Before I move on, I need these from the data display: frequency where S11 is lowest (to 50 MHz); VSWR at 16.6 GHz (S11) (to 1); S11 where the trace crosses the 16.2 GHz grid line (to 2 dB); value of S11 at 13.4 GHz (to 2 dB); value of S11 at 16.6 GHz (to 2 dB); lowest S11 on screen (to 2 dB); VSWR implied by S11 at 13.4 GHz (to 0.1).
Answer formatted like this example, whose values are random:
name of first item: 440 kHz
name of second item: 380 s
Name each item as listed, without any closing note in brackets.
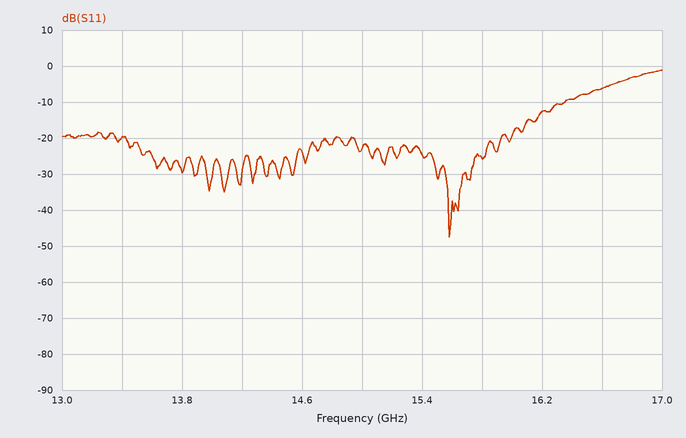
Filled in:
frequency where S11 is lowest: 15.60 GHz
VSWR at 16.6 GHz (S11): 3
S11 where the trace crosses the 16.2 GHz grid line: -12 dB
value of S11 at 13.4 GHz: -20 dB
value of S11 at 16.6 GHz: -6 dB
lowest S11 on screen: -48 dB
VSWR implied by S11 at 13.4 GHz: 1.2
